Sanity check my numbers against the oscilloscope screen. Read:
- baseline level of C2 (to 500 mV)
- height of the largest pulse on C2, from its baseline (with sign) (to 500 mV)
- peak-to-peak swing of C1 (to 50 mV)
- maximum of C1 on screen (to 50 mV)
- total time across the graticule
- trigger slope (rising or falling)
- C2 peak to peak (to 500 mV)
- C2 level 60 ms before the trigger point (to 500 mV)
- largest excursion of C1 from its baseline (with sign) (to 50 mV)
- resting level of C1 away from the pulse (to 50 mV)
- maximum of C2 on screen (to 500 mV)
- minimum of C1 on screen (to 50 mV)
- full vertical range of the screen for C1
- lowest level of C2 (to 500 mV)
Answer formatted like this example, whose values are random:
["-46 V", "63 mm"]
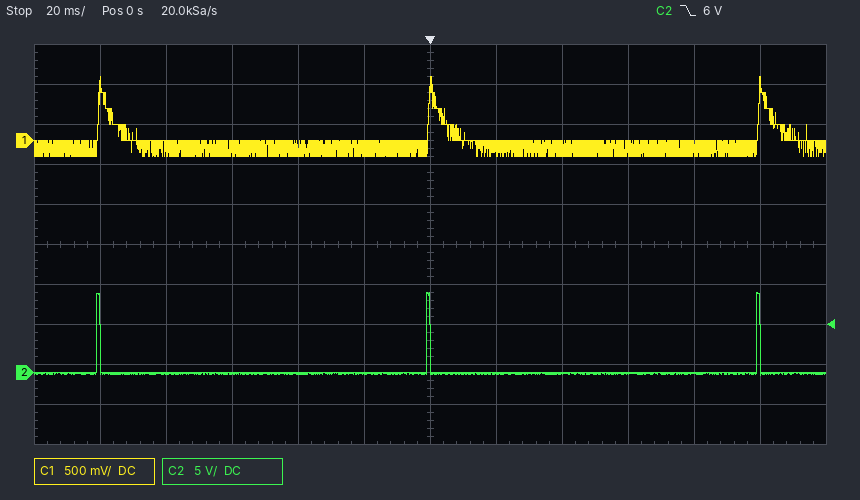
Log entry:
["0.0 V", "+10.0 V", "1.00 V", "800 mV", "240 ms", "falling", "10.5 V", "0.0 V", "+900 mV", "-100 mV", "10.0 V", "-200 mV", "5 V", "-500 mV"]
